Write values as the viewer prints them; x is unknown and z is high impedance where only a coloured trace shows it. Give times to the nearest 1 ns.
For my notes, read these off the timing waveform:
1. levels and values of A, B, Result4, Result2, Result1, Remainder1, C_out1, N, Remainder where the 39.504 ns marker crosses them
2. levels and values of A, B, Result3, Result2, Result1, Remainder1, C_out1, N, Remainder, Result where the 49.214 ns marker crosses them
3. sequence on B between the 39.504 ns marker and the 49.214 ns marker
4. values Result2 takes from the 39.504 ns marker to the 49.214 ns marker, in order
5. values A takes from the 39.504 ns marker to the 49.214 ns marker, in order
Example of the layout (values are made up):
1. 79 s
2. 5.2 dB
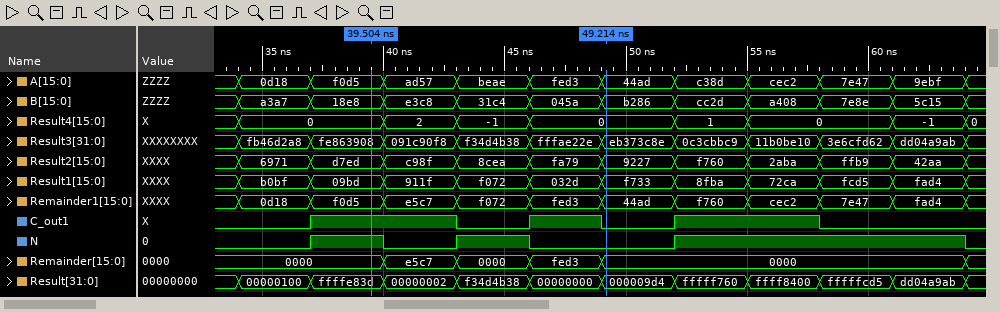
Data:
1. A=f0d5, B=18e8, Result4=0, Result2=d7ed, Result1=09bd, Remainder1=f0d5, C_out1=1, N=1, Remainder=0000
2. A=44ad, B=b286, Result3=eb373c8e, Result2=9227, Result1=f733, Remainder1=44ad, C_out1=0, N=0, Remainder=0000, Result=000009d4
3. 18e8, e3c8, 31c4, 045a, b286
4. d7ed, c98f, 8cea, fa79, 9227
5. f0d5, ad57, beae, fed3, 44ad
